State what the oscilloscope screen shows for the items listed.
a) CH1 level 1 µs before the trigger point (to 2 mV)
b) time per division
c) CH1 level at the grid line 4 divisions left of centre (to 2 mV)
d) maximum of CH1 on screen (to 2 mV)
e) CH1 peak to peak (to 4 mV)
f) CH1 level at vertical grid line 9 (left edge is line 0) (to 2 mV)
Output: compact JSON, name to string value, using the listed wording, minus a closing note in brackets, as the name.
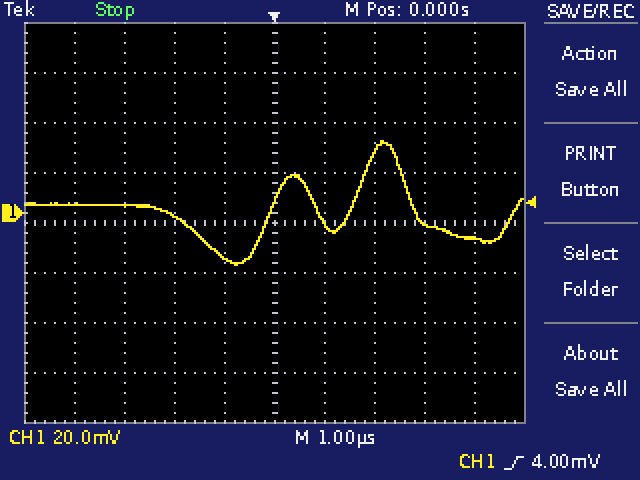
{"CH1 level 1 µs before the trigger point": "-18 mV", "time per division": "1 µs", "CH1 level at the grid line 4 divisions left of centre": "4 mV", "maximum of CH1 on screen": "28 mV", "CH1 peak to peak": "48 mV", "CH1 level at vertical grid line 9 (left edge is line 0)": "-10 mV"}
